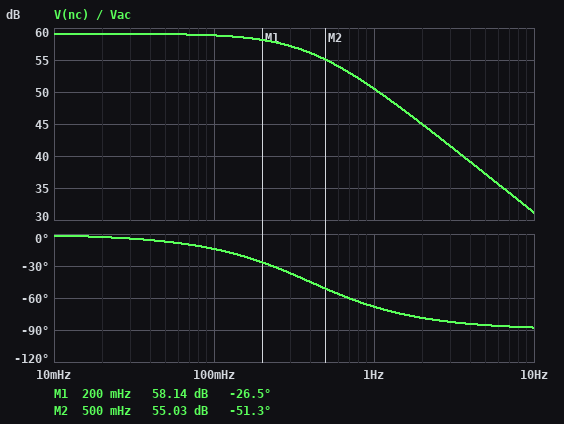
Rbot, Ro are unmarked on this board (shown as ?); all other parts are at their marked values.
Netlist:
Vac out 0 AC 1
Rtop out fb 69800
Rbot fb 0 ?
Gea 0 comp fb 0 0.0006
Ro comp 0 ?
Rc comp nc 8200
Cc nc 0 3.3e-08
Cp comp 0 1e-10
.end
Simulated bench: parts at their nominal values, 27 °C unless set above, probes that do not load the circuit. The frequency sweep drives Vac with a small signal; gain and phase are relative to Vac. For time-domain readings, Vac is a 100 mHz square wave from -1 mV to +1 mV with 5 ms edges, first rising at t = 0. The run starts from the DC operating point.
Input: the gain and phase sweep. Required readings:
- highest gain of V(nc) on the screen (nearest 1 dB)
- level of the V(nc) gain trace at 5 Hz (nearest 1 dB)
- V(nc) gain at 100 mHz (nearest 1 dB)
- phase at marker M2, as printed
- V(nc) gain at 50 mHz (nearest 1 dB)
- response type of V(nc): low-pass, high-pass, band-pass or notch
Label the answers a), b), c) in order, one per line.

a) 59 dB
b) 37 dB
c) 59 dB
d) -51.3 deg
e) 59 dB
f) low-pass
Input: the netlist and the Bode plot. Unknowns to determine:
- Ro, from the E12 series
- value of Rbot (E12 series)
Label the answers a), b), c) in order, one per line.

a) 12 MΩ
b) 10 kΩ
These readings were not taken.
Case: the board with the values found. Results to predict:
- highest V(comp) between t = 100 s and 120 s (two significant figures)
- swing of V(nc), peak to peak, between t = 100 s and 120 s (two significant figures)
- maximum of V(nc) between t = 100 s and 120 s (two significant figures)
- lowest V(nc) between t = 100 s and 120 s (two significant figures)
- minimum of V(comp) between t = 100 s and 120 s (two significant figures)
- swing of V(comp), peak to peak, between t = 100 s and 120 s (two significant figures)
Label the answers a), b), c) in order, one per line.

a) 900 mV
b) 1.8 V
c) 900 mV
d) -900 mV
e) -900 mV
f) 1.8 V
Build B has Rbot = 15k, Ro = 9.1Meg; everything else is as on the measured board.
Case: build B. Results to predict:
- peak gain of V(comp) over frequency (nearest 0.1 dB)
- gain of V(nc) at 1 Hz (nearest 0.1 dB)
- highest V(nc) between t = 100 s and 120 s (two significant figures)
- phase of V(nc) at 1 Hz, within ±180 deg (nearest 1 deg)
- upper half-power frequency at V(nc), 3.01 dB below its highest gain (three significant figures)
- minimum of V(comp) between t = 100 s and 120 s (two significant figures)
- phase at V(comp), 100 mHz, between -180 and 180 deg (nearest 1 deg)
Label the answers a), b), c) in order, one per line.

a) 59.7 dB
b) 53.1 dB
c) 970 mV
d) -62 deg
e) 528 mHz
f) -970 mV
g) -11 deg
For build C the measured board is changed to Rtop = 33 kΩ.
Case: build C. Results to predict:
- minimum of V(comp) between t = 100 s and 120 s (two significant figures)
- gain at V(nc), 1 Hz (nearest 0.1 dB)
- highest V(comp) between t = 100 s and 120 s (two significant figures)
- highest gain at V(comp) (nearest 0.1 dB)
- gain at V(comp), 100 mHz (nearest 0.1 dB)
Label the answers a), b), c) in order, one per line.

a) -1.7 V
b) 55.9 dB
c) 1.7 V
d) 64.5 dB
e) 64.2 dB
